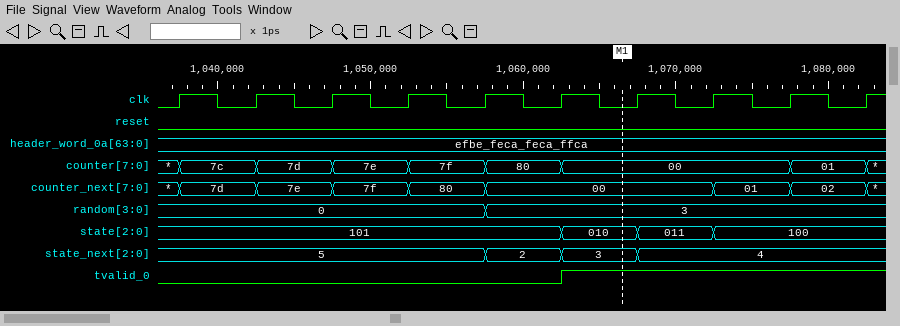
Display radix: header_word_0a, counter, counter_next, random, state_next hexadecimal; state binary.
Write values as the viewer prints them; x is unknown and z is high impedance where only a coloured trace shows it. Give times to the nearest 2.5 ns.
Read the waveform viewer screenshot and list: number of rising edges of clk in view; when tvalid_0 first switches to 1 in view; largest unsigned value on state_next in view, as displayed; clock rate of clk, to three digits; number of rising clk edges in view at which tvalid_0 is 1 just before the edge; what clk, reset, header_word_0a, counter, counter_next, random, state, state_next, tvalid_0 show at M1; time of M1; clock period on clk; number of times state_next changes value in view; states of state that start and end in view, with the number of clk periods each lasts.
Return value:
10
1062.5 ns
5
200 MHz
4
clk=0, reset=0, header_word_0a=efbe_feca_feca_ffca, counter=00, counter_next=00, random=3, state=010, state_next=3, tvalid_0=1
1067.5 ns
5 ns
3
010: 1, 011: 1
